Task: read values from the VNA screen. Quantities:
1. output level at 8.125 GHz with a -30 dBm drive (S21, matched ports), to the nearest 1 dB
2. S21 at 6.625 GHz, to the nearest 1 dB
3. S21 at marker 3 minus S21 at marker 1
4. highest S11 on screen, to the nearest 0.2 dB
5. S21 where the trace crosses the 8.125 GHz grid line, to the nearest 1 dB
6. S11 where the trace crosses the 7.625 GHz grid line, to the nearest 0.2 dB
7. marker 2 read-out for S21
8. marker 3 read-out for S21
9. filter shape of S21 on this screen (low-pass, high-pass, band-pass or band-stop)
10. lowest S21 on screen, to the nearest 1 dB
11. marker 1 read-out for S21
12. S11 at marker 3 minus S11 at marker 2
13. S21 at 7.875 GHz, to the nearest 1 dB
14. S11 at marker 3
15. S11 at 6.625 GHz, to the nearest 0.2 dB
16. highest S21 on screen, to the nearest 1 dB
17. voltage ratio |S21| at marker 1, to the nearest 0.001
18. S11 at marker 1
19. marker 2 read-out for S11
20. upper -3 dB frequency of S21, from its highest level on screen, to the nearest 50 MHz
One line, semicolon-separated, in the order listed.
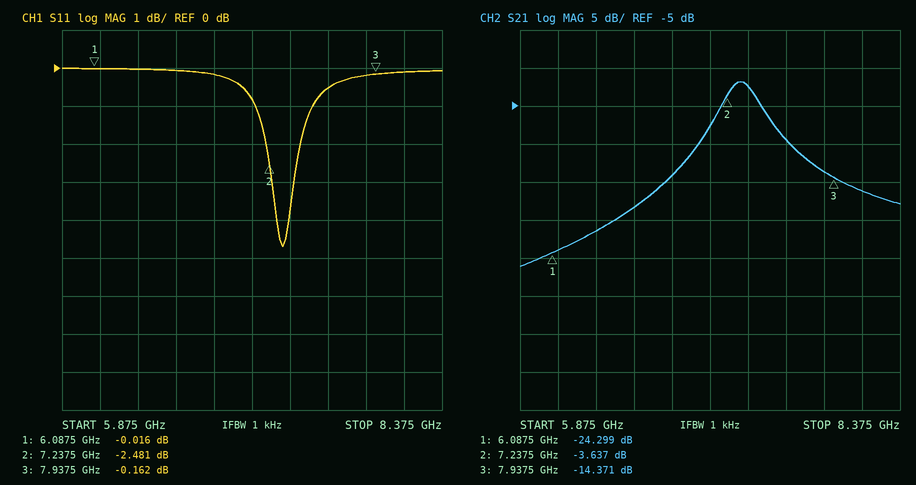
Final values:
-46 dBm; -18 dB; 9.928 dB; 0.0 dB; -16 dB; -0.6 dB; -3.637 dB; -14.371 dB; band-pass; -26 dB; -24.299 dB; 2.319 dB; -14 dB; -0.162 dB; 0.0 dB; -2 dB; 0.061; -0.016 dB; -2.481 dB; 7.45 GHz
